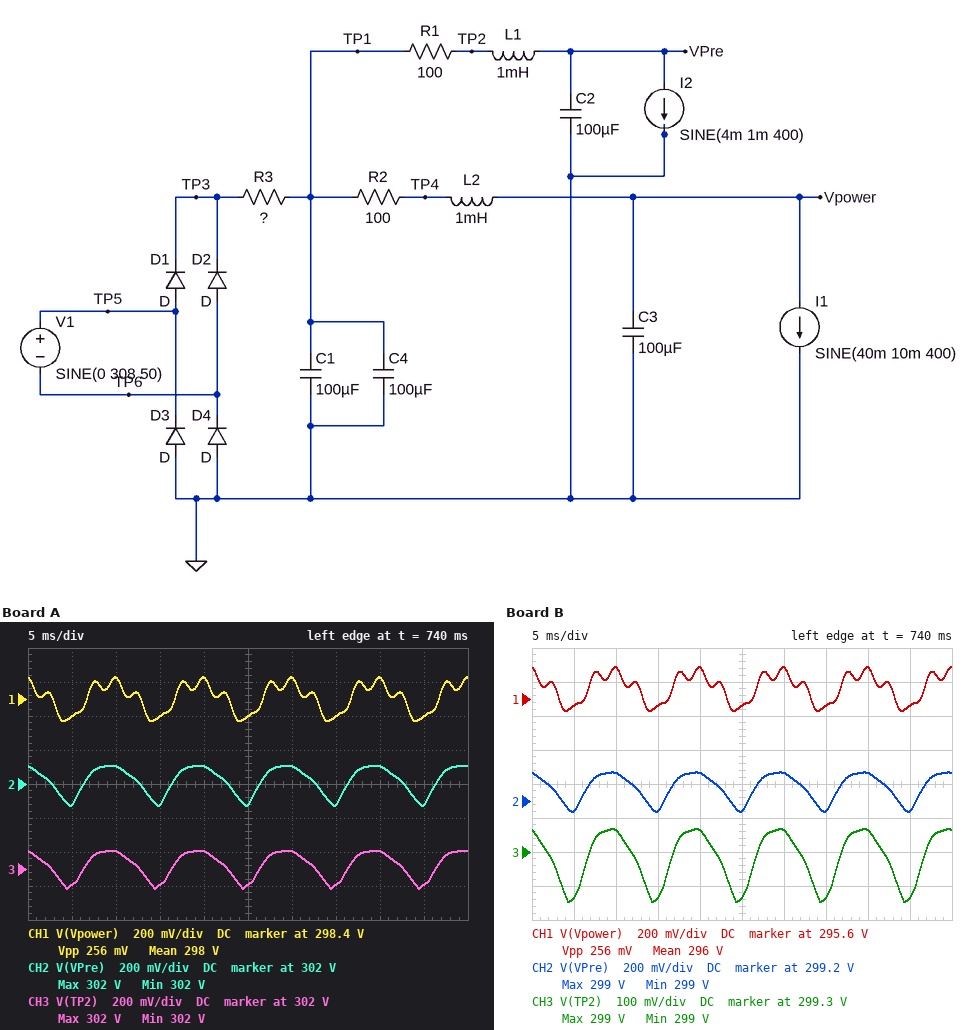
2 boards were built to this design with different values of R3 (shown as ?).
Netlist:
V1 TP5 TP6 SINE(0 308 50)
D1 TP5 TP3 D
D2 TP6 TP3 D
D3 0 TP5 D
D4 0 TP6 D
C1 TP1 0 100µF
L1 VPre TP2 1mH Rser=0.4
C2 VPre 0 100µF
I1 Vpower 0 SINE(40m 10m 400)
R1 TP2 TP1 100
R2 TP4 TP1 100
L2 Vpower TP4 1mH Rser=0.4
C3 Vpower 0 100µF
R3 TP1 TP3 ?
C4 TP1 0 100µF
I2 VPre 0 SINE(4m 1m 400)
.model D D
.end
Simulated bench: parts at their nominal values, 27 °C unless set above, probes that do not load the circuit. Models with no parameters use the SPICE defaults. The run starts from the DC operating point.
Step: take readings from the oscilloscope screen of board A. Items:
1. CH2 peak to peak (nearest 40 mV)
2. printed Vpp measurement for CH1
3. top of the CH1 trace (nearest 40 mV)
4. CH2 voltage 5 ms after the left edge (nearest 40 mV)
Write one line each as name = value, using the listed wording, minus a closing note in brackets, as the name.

CH2 peak to peak = 240 mV
printed Vpp measurement for CH1 = 256 mV
top of the CH1 trace = 298.52 V
CH2 voltage 5 ms after the left edge = 301.88 V
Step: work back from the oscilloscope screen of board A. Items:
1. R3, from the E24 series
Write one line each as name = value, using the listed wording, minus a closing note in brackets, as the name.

R3, from the E24 series = 5.6 Ω
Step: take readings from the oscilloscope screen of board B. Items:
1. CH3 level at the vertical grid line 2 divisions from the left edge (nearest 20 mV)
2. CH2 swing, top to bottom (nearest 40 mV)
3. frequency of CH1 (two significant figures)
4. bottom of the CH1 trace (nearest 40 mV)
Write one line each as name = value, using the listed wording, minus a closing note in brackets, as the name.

CH3 level at the vertical grid line 2 divisions from the left edge = 299.36 V
CH2 swing, top to bottom = 240 mV
frequency of CH1 = 100 Hz
bottom of the CH1 trace = 295.52 V
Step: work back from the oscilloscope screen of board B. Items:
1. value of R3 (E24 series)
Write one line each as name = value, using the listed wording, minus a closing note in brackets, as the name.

value of R3 = 13 Ω
